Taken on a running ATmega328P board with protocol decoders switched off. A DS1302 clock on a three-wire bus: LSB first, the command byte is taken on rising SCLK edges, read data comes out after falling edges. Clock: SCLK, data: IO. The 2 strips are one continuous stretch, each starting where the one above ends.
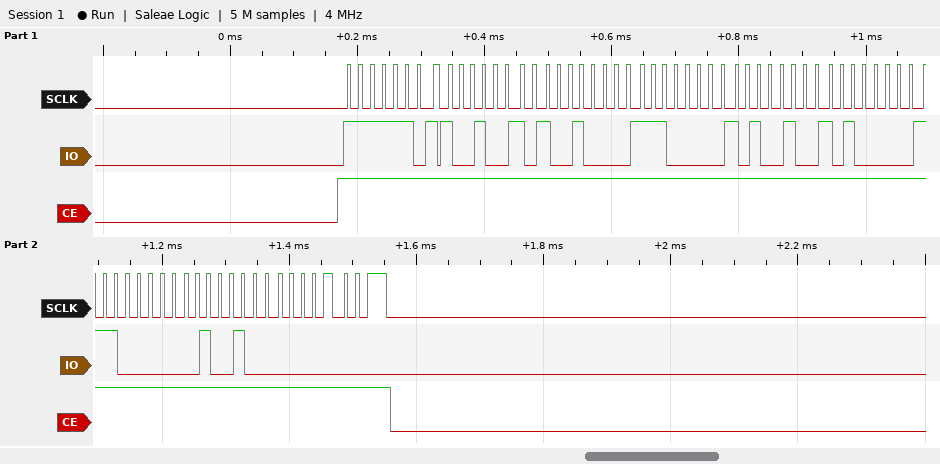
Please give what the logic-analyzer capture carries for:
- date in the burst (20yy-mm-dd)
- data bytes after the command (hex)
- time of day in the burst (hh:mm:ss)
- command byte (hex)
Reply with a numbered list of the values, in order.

1. 2024-05-25
2. 49 09 07 25 05 07 24 00
3. 07:09:49
4. 0xBF
